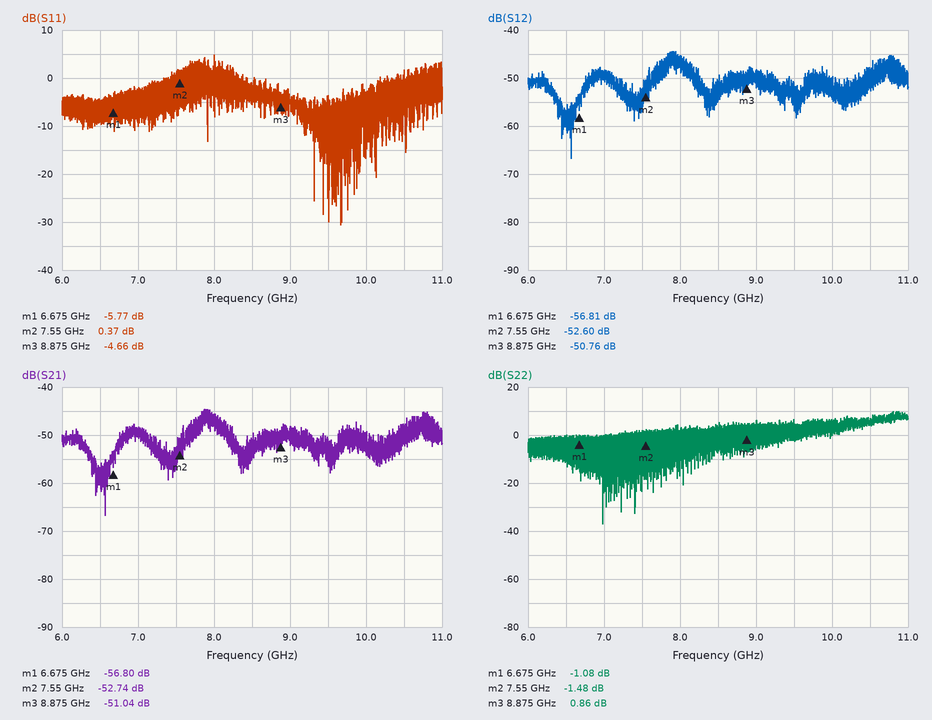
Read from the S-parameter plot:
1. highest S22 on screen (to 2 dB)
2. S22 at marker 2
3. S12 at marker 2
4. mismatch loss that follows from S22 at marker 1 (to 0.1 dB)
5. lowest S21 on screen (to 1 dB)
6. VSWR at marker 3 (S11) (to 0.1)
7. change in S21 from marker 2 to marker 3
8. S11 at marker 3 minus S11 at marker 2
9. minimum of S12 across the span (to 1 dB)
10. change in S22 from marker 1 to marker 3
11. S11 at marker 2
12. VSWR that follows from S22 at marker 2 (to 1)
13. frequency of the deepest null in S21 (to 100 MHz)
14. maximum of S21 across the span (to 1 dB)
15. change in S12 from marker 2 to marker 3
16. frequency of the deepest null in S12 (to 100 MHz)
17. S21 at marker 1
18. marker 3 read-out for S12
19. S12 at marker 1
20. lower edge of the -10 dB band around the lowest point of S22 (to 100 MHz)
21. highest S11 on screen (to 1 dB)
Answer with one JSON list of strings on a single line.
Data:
["10 dB", "-1.48 dB", "-52.60 dB", "6.6 dB", "-67 dB", "3.8", "1.70 dB", "-5.03 dB", "-67 dB", "1.94 dB", "0.37 dB", "12", "6.6 GHz", "-45 dB", "1.84 dB", "6.6 GHz", "-56.80 dB", "-50.76 dB", "-56.81 dB", "7.0 GHz", "5 dB"]
